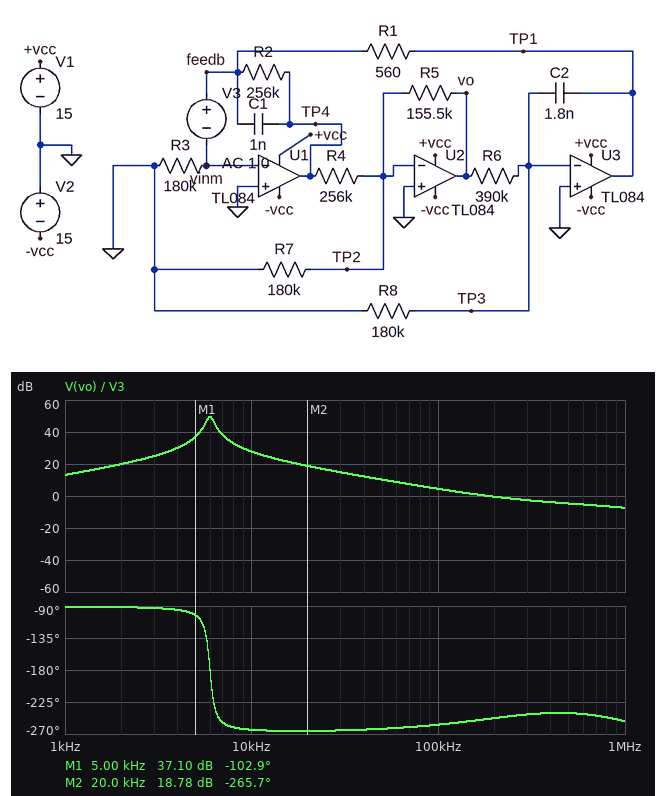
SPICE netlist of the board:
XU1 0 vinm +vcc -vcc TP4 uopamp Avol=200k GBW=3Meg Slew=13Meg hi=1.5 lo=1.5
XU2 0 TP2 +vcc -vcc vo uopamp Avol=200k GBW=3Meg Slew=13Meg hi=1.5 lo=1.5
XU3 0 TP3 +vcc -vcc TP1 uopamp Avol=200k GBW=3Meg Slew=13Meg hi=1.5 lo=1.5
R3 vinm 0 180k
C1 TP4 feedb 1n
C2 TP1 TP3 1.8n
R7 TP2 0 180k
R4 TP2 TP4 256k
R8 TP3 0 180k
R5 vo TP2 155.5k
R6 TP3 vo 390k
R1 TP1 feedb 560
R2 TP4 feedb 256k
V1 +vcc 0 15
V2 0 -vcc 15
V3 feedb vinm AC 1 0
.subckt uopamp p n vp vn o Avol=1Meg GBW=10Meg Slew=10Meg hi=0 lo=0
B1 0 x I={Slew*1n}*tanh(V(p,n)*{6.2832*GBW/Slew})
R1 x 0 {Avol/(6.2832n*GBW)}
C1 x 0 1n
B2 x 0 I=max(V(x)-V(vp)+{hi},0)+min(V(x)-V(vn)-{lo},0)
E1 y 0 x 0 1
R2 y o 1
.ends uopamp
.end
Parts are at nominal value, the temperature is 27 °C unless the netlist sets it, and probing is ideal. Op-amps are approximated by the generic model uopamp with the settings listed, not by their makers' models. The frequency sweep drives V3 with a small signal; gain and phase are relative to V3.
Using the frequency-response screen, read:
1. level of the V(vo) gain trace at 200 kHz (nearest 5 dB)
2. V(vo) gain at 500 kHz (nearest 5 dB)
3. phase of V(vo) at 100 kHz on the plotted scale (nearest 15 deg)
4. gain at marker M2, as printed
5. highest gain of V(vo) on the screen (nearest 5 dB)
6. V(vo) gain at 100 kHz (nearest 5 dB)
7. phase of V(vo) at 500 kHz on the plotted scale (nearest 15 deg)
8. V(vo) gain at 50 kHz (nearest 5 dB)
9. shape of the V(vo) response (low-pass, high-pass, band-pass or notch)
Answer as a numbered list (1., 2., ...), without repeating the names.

1. 0 dB
2. -5 dB
3. -255 deg
4. 18.78 dB
5. 50 dB
6. 5 dB
7. -240 deg
8. 10 dB
9. band-pass
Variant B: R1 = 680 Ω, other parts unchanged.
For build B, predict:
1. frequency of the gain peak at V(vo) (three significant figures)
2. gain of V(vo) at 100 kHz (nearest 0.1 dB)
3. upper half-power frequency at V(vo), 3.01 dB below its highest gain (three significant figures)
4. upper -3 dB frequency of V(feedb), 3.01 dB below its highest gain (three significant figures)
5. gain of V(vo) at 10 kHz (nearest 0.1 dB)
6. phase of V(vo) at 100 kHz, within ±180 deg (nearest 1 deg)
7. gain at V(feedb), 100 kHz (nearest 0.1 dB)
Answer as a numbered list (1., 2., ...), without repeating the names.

1. 5.47 kHz
2. 3.1 dB
3. 5.74 kHz
4. 5.57 kHz
5. 25.5 dB
6. 107 deg
7. -0.7 dB
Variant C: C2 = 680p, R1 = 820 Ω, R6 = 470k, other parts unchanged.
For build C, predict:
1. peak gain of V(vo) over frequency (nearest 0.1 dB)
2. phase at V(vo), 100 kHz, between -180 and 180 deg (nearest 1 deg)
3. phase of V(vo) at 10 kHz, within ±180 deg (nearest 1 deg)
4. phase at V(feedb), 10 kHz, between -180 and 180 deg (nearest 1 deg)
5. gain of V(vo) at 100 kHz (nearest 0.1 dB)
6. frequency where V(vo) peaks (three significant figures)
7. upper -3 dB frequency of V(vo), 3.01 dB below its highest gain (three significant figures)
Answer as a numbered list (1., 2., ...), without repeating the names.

1. 46.9 dB
2. 111 deg
3. 99 deg
4. -1 deg
5. 1.9 dB
6. 7.42 kHz
7. 7.68 kHz
